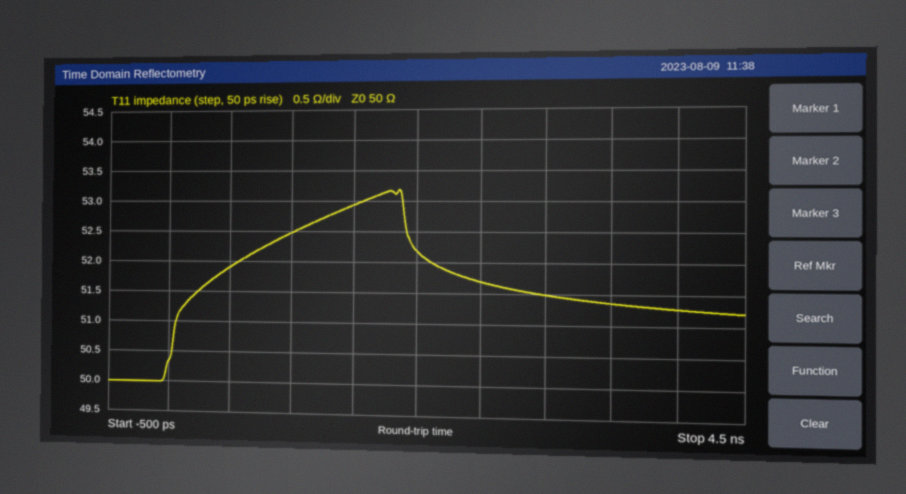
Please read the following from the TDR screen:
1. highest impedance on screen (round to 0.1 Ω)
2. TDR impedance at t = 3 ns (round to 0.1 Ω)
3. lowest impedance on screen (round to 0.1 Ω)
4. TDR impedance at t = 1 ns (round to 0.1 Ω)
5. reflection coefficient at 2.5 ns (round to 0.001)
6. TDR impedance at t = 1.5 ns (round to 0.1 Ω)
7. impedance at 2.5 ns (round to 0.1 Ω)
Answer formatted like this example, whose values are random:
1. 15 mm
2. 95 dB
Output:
1. 53.2 Ω
2. 51.5 Ω
3. 50.0 Ω
4. 52.5 Ω
5. +0.017
6. 52.9 Ω
7. 51.7 Ω
